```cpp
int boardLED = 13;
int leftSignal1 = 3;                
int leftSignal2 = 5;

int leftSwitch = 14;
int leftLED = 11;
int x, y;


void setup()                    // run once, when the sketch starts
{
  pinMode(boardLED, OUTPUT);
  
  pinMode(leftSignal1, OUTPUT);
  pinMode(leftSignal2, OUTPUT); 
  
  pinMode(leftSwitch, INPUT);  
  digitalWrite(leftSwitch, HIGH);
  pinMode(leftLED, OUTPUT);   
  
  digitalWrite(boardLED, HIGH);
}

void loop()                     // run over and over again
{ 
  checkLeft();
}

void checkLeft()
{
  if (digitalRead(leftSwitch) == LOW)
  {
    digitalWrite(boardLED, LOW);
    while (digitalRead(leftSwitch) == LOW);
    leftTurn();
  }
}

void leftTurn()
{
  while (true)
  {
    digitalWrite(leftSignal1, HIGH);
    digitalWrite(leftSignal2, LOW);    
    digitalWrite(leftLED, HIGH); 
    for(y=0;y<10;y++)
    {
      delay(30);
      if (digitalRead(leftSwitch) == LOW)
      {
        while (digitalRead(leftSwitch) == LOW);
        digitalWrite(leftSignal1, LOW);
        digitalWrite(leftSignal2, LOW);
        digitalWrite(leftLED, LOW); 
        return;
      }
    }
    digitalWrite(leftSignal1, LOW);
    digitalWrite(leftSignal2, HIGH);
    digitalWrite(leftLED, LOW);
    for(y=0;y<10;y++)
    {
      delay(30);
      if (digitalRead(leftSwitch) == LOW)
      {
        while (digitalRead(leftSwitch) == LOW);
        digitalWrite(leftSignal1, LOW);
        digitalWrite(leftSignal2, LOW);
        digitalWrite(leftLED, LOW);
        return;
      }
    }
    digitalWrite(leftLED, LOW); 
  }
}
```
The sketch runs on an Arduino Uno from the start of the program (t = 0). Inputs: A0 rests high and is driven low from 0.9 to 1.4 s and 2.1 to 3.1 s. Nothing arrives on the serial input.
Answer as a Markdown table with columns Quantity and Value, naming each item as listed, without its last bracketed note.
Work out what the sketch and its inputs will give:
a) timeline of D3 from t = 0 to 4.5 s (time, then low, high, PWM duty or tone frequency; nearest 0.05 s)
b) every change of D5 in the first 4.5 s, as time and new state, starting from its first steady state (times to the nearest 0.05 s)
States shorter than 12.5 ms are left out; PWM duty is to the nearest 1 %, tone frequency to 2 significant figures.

| Quantity | Value |
|---|---|
| timeline of D3 from t = 0 to 4.5 s | 0 s low; 1.4 s high; 1.7 s low; 2 s high; 3.1 s low |
| every change of D5 in the first 4.5 s, as time and new state, starting from its first steady state | 0 s low; 1.7 s high; 2 s low |
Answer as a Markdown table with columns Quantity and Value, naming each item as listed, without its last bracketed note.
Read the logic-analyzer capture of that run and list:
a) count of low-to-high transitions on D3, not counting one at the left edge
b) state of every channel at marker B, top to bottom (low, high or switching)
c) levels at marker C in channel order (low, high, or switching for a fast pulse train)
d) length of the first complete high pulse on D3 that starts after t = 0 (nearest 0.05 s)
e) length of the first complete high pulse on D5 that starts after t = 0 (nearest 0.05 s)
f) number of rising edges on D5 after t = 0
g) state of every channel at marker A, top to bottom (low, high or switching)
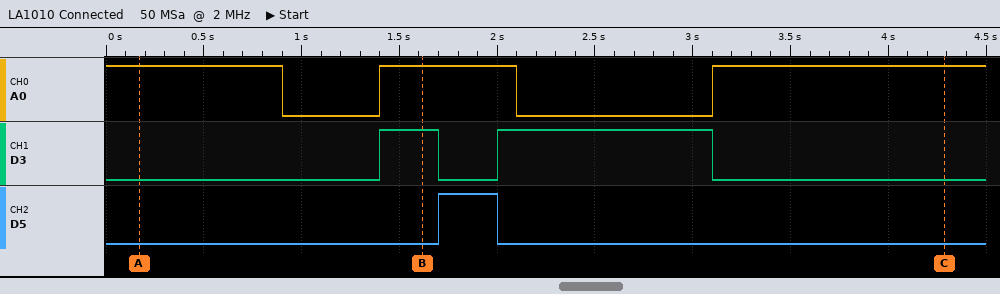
| Quantity | Value |
|---|---|
| count of low-to-high transitions on D3, not counting one at the left edge | 2 |
| state of every channel at marker B, top to bottom | A0 high, D3 high, D5 low |
| levels at marker C in channel order | A0 high, D3 low, D5 low |
| length of the first complete high pulse on D3 that starts after t = 0 | 0.30 s |
| length of the first complete high pulse on D5 that starts after t = 0 | 0.30 s |
| number of rising edges on D5 after t = 0 | 1 |
| state of every channel at marker A, top to bottom | A0 high, D3 low, D5 low |
